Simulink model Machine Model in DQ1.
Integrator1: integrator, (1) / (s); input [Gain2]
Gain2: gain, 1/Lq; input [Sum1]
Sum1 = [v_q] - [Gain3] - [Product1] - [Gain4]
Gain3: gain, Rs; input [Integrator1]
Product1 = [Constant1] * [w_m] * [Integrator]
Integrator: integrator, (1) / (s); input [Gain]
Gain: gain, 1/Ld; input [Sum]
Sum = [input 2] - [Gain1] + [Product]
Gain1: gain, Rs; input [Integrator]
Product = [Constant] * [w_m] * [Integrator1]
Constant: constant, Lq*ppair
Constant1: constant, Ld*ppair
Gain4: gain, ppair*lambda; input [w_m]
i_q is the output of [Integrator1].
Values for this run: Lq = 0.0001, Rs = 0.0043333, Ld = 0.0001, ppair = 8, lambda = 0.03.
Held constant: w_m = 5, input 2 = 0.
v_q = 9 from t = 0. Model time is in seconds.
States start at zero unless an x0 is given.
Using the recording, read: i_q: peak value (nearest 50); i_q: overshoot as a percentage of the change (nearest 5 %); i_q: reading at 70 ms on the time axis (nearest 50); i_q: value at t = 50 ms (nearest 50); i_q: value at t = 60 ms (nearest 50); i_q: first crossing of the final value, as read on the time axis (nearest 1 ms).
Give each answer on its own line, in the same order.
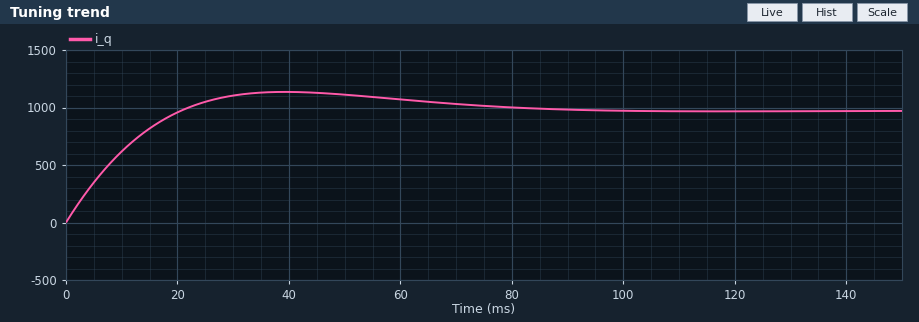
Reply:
1150
15 %
1050
1100
1050
21 ms
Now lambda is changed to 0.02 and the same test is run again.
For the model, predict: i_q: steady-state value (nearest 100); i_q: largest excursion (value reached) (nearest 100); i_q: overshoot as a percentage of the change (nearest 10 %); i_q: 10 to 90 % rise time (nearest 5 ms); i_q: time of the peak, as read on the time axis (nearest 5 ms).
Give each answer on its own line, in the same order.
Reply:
1000
1200
20 %
15 ms
40 ms
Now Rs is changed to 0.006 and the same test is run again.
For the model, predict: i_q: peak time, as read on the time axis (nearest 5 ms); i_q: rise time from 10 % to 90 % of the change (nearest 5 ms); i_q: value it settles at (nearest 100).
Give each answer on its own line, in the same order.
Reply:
40 ms
15 ms
900
